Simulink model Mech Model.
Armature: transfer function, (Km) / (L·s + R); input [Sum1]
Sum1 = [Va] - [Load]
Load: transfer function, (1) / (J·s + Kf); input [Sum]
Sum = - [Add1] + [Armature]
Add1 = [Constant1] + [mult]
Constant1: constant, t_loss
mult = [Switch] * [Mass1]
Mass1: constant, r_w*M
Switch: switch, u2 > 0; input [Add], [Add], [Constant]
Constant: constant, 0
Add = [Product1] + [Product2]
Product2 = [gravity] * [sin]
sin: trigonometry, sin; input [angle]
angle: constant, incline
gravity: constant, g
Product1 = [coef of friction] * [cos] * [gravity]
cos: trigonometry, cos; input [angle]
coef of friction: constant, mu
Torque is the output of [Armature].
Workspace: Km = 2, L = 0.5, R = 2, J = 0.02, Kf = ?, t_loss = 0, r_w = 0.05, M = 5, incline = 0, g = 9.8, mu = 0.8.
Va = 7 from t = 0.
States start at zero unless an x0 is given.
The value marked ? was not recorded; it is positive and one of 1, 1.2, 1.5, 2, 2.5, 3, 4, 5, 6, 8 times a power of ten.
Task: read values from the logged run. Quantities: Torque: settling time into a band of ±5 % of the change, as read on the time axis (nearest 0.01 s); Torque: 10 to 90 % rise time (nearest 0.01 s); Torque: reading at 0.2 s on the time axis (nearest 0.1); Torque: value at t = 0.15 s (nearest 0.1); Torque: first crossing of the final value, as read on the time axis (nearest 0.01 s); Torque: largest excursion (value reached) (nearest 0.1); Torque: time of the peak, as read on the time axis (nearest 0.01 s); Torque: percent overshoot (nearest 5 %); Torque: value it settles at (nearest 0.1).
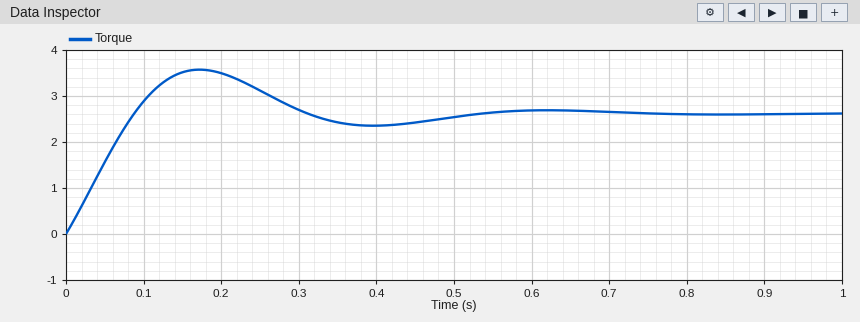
0.48 s
0.07 s
3.5
3.5
0.09 s
3.6
0.17 s
35 %
2.6
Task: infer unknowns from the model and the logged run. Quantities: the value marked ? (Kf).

0.15
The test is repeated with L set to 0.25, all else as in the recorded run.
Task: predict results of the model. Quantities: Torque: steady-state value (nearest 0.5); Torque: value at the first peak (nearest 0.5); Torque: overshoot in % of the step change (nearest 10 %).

2.5
4.0
50 %
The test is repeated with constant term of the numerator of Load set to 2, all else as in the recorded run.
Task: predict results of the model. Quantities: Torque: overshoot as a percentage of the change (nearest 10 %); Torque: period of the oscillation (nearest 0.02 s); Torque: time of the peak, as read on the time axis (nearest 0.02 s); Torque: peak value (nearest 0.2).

50 %
0.32 s
0.12 s
3.4
